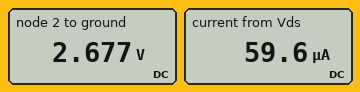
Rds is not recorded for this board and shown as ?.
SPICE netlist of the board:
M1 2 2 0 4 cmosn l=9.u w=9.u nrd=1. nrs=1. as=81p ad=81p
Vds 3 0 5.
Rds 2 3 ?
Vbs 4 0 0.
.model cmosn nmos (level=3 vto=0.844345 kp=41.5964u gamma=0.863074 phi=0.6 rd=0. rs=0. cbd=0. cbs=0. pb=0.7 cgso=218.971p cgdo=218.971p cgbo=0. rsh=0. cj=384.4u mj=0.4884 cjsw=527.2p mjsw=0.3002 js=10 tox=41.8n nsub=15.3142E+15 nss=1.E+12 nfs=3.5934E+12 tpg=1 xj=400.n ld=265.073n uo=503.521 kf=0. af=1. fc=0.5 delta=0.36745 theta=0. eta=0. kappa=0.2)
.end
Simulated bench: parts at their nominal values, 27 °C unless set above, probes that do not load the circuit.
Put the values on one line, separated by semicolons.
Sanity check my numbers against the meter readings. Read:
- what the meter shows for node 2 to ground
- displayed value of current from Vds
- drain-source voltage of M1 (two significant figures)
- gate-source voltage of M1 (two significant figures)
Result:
2.677 V; 59.6 µA; 2.7 V; 2.7 V
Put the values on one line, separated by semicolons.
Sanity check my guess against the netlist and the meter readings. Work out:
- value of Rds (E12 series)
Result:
39 kΩ
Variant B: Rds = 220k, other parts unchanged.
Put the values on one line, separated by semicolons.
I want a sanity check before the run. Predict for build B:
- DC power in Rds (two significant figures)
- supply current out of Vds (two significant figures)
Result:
48 µW; 15 µA
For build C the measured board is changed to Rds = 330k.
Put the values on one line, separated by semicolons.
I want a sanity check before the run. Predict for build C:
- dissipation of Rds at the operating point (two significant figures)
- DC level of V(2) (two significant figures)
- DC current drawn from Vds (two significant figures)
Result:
35 µW; 1.6 V; 10 µA
